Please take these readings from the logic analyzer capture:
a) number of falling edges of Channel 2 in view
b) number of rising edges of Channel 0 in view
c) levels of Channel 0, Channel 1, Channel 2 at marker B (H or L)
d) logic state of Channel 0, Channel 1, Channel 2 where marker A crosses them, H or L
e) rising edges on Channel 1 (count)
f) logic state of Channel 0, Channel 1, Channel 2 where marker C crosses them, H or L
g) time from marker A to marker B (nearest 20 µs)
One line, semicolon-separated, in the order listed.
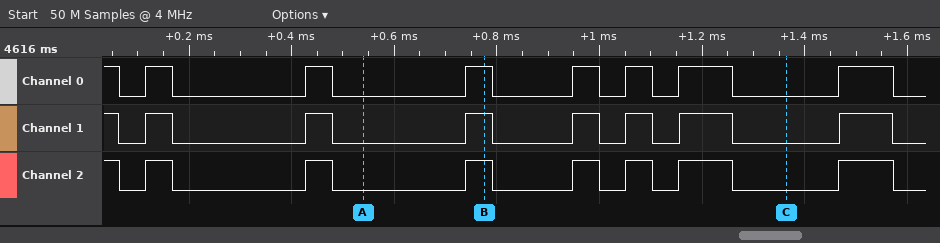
8; 7; Channel 0=H, Channel 1=H, Channel 2=H; Channel 0=L, Channel 1=L, Channel 2=L; 7; Channel 0=L, Channel 1=L, Channel 2=L; 240 µs
